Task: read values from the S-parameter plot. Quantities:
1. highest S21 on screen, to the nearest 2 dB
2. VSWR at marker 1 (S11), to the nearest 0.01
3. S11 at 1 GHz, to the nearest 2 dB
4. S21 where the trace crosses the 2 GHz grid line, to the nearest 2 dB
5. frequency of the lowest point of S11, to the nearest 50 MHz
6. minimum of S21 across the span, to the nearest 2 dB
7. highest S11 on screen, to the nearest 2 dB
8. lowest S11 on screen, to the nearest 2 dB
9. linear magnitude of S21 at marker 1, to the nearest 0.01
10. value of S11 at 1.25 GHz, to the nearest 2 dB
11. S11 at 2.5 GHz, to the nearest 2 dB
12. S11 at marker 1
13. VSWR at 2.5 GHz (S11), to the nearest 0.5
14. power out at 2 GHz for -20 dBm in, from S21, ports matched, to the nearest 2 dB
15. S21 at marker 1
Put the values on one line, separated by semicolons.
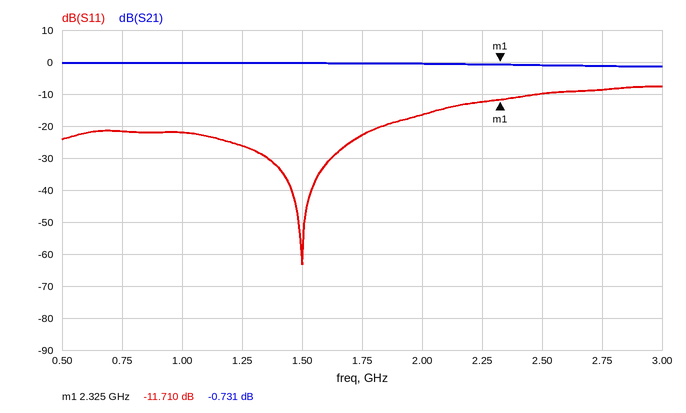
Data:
0 dB; 1.70; -22 dB; 0 dB; 1.50 GHz; -2 dB; -8 dB; -64 dB; 0.92; -26 dB; -10 dB; -11.710 dB; 2.0; -20 dBm; -0.731 dB
